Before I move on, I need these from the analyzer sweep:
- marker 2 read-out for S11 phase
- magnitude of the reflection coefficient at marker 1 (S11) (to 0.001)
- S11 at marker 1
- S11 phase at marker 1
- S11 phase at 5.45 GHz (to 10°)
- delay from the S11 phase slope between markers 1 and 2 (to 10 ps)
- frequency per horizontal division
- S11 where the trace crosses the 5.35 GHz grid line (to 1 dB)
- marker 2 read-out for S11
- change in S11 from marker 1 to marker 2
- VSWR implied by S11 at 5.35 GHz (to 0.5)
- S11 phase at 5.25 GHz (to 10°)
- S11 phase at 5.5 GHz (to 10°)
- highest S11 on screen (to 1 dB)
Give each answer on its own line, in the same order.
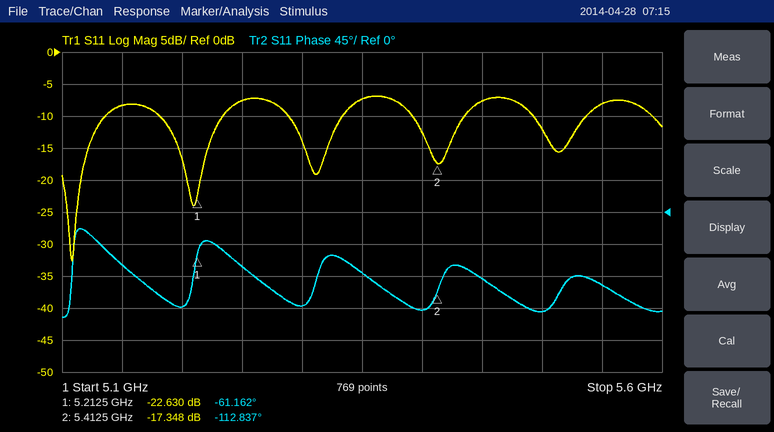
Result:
-112.837°
0.074
-22.630 dB
-61.162°
-90°
720 ps
50 MHz
-7 dB
-17.348 dB
5.282 dB
2.5
-80°
-140°
-7 dB
